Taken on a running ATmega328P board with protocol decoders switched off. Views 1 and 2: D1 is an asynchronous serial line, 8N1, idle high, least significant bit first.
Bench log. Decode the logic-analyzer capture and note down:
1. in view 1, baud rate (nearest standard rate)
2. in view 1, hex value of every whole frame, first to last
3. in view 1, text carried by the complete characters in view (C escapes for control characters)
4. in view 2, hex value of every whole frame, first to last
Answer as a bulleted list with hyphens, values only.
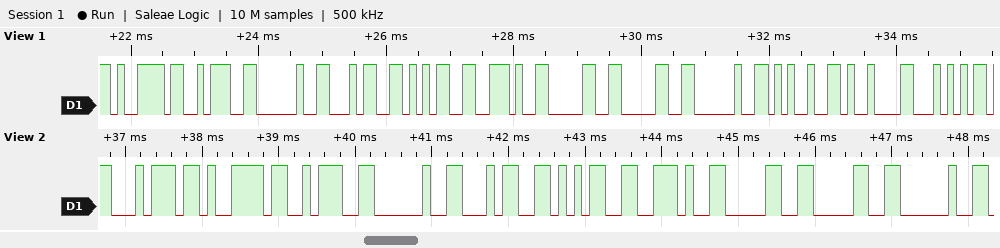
- 9600 baud
- 0x79 0x3A 0x20 0x34 0x35 0x2E 0x30 0x30 0x20 0x25 0x09 0x54
- "y: 45.00 %\tT"
- 74 79 3A 20 34 35 2E 30 30 20
